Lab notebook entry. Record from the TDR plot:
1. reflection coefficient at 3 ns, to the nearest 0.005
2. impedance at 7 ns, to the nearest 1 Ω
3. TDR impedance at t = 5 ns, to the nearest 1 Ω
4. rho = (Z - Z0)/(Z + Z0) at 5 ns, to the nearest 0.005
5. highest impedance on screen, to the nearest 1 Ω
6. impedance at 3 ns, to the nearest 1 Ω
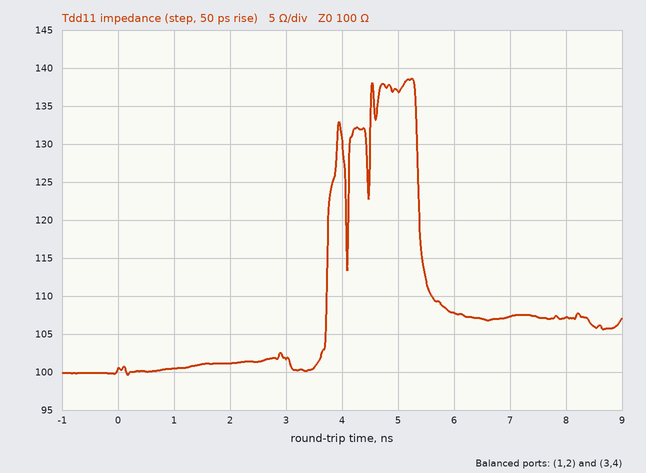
+0.010
107 Ω
137 Ω
+0.155
139 Ω
102 Ω
